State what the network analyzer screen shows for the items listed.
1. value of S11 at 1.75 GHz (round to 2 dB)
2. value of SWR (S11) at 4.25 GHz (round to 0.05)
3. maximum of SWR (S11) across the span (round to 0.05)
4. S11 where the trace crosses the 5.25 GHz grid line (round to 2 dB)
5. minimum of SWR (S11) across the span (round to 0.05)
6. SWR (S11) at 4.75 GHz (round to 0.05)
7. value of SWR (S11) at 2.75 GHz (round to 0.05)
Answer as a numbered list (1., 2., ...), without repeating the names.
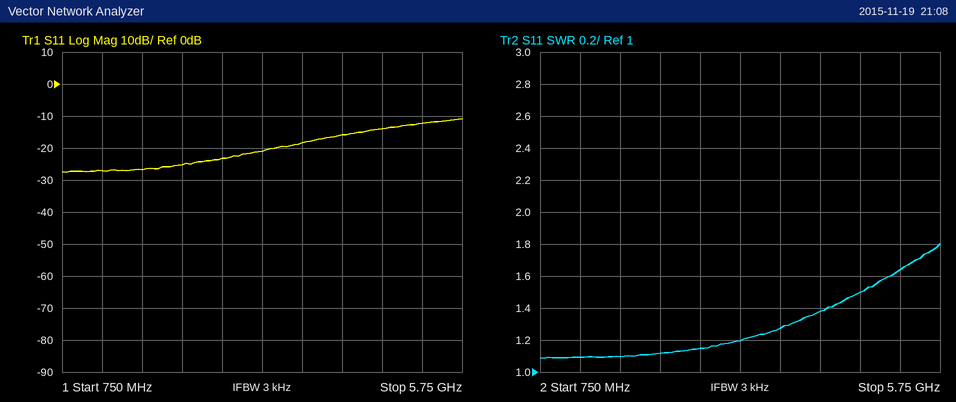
1. -26 dB
2. 1.40
3. 1.80
4. -12 dB
5. 1.10
6. 1.50
7. 1.15
